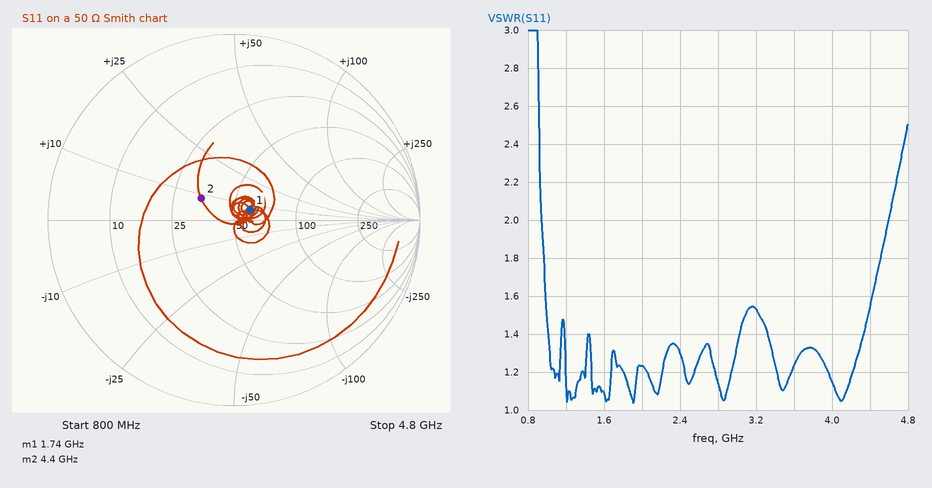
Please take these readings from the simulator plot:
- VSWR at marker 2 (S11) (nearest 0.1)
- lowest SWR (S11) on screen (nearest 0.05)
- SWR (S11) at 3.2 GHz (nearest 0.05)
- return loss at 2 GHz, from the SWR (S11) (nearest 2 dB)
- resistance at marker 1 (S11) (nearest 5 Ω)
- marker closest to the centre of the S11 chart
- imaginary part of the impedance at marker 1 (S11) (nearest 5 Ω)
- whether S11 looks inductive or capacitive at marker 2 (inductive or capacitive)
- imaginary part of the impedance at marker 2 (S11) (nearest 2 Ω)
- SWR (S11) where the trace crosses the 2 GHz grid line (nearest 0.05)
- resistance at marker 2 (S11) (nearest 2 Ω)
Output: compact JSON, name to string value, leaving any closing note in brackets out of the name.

{"VSWR at marker 2 (S11)": "1.5", "lowest SWR (S11) on screen": "1.05", "SWR (S11) at 3.2 GHz": "1.55", "return loss at 2 GHz, from the SWR (S11)": "20 dB", "resistance at marker 1 (S11)": "60 Ω", "marker closest to the centre of the S11 chart": "marker 1", "imaginary part of the impedance at marker 1 (S11)": "+5 Ω", "whether S11 looks inductive or capacitive at marker 2": "inductive", "imaginary part of the impedance at marker 2 (S11)": "+8 Ω", "SWR (S11) where the trace crosses the 2 GHz grid line": "1.25", "resistance at marker 2 (S11)": "34 Ω"}
